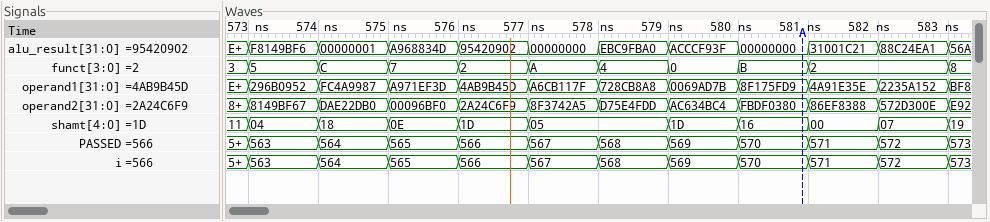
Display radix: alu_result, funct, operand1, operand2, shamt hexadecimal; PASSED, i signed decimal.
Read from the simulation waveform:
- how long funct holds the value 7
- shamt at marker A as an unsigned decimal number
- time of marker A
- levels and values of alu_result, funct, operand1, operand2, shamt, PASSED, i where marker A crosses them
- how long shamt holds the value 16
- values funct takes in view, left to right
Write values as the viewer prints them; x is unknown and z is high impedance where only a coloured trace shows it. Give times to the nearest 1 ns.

1 ns
22
581 ns
alu_result=00000000, funct=B, operand1=8F175FD9, operand2=FBDF0380, shamt=16, PASSED=570, i=570
1 ns
3, 5, C, 7, 2, A, 4, 0, B, 2, 8
